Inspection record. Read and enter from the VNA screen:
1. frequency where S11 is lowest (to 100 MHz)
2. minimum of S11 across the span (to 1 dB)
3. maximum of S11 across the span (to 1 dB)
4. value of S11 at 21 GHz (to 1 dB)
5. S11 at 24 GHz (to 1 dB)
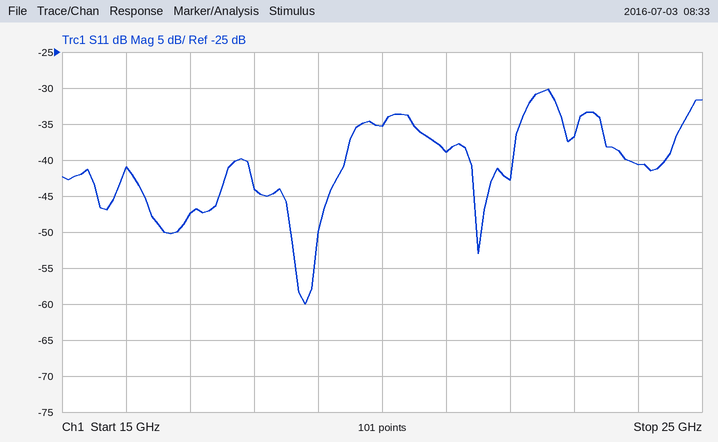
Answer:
18.8 GHz
-60 dB
-30 dB
-39 dB
-41 dB
